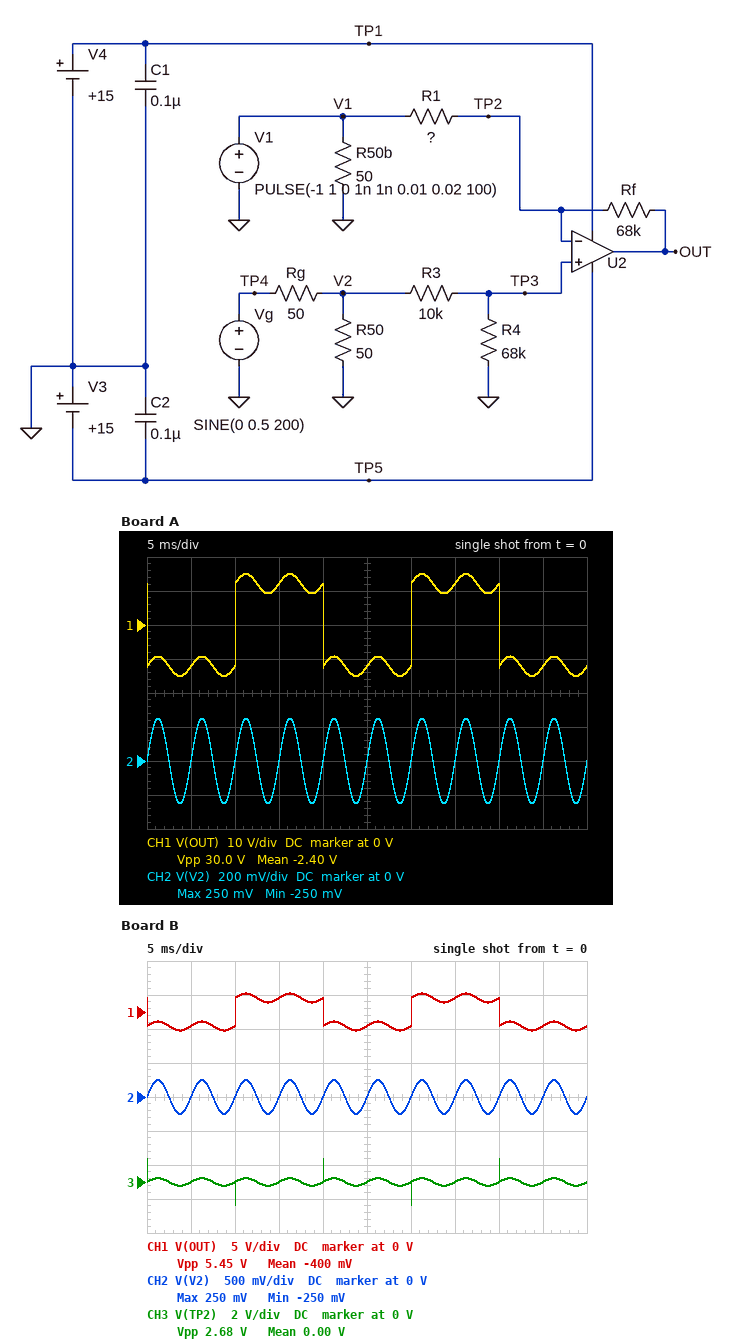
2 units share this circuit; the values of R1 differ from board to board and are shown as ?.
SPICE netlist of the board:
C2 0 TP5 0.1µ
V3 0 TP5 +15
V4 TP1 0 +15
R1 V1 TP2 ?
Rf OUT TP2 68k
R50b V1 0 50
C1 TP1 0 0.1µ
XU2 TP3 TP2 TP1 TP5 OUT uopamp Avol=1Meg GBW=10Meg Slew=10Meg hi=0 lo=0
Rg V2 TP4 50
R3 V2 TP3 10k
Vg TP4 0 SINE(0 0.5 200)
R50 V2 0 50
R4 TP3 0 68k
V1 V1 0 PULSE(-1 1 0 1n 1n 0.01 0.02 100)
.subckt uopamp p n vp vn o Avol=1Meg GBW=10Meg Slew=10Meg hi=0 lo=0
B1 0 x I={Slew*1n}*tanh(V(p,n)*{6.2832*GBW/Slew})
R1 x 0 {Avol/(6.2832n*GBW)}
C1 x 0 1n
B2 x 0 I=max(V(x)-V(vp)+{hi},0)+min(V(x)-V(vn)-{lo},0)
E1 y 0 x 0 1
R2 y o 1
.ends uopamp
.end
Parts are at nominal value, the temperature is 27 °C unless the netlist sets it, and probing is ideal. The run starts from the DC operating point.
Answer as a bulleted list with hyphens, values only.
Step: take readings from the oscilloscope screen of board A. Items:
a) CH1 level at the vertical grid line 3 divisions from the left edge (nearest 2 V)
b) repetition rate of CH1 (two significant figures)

- 12 V
- 50 Hz
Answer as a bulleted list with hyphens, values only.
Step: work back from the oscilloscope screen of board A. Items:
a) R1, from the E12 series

- 5.6 kΩ
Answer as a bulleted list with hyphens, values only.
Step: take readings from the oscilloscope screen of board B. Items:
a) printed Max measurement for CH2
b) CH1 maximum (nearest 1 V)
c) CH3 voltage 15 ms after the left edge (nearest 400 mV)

- 250 mV
- 3 V
- 0 V
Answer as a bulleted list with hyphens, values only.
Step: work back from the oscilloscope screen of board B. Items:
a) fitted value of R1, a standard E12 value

- 33 kΩ
